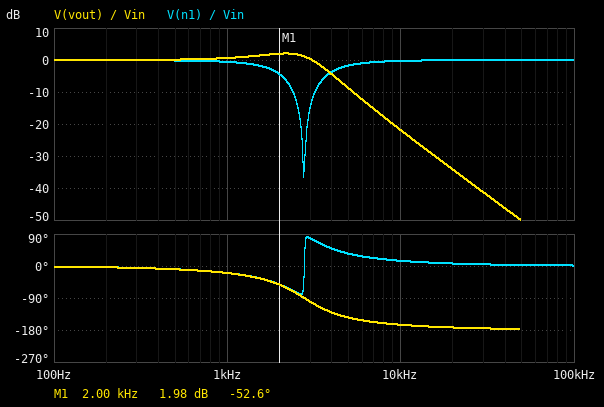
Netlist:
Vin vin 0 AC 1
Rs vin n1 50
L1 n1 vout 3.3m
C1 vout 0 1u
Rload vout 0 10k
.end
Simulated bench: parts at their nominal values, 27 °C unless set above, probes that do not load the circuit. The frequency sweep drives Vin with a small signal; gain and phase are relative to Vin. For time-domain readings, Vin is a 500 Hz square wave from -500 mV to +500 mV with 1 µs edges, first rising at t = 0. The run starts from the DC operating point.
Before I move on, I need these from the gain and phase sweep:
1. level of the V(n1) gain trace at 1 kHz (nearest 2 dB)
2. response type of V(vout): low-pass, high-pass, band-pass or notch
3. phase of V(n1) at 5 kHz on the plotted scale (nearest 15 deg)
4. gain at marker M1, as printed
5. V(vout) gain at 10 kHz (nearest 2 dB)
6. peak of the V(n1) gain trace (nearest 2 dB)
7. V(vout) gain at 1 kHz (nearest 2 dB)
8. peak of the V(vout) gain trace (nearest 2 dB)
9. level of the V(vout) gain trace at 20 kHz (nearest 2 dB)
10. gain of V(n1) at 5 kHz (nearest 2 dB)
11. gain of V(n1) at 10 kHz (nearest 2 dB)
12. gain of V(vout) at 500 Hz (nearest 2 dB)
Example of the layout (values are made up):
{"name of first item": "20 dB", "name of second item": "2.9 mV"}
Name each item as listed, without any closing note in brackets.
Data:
{"level of the V(n1) gain trace at 1 kHz": "0 dB", "response type of V(vout): low-pass, high-pass, band-pass or notch": "low-pass", "phase of V(n1) at 5 kHz on the plotted scale": "30 deg", "gain at marker M1, as printed": "1.98 dB", "V(vout) gain at 10 kHz": "-22 dB", "peak of the V(n1) gain trace": "0 dB", "V(vout) gain at 1 kHz": "0 dB", "peak of the V(vout) gain trace": "2 dB", "level of the V(vout) gain trace at 20 kHz": "-34 dB", "gain of V(n1) at 5 kHz": "-2 dB", "gain of V(n1) at 10 kHz": "0 dB", "gain of V(vout) at 500 Hz": "0 dB"}
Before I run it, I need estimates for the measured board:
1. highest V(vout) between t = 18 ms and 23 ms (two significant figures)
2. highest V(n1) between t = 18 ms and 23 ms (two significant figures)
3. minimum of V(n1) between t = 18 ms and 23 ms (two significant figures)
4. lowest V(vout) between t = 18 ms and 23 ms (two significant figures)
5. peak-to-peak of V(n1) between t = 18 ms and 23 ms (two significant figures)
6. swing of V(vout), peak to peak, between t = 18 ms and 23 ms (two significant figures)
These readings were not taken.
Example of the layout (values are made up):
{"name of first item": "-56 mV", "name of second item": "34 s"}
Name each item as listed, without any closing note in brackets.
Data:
{"highest V(vout) between t = 18 ms and 23 ms": "710 mV", "highest V(n1) between t = 18 ms and 23 ms": "610 mV", "minimum of V(n1) between t = 18 ms and 23 ms": "-610 mV", "lowest V(vout) between t = 18 ms and 23 ms": "-710 mV", "peak-to-peak of V(n1) between t = 18 ms and 23 ms": "1.2 V", "swing of V(vout), peak to peak, between t = 18 ms and 23 ms": "1.4 V"}
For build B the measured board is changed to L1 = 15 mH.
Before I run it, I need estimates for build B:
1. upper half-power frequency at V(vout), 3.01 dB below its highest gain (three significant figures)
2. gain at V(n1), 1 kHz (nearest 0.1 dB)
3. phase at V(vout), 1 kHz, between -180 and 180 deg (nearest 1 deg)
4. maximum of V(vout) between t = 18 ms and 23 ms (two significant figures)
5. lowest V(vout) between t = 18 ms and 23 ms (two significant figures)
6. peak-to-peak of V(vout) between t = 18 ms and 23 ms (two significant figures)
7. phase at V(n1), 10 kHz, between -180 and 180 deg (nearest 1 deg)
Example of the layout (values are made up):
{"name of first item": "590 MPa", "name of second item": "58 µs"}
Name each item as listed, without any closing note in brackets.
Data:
{"upper half-power frequency at V(vout), 3.01 dB below its highest gain": "1.50 kHz", "gain at V(n1), 1 kHz": "-2.2 dB", "phase at V(vout), 1 kHz, between -180 and 180 deg": "-38 deg", "maximum of V(vout) between t = 18 ms and 23 ms": "990 mV", "lowest V(vout) between t = 18 ms and 23 ms": "-990 mV", "peak-to-peak of V(vout) between t = 18 ms and 23 ms": "2.0 V", "phase at V(n1), 10 kHz, between -180 and 180 deg": "3 deg"}
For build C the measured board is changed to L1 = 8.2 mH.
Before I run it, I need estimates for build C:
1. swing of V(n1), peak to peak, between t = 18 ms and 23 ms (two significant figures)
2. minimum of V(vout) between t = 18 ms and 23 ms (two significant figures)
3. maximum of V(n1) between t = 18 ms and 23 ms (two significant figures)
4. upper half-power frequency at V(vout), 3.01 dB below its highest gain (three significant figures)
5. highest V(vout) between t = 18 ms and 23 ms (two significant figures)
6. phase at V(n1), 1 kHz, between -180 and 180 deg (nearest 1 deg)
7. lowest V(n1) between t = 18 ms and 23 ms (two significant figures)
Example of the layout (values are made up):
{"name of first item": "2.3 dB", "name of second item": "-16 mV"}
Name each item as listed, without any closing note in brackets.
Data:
{"swing of V(n1), peak to peak, between t = 18 ms and 23 ms": "1.3 V", "minimum of V(vout) between t = 18 ms and 23 ms": "-910 mV", "maximum of V(n1) between t = 18 ms and 23 ms": "650 mV", "upper half-power frequency at V(vout), 3.01 dB below its highest gain": "2.07 kHz", "highest V(vout) between t = 18 ms and 23 ms": "910 mV", "phase at V(n1), 1 kHz, between -180 and 180 deg": "-25 deg", "lowest V(n1) between t = 18 ms and 23 ms": "-650 mV"}
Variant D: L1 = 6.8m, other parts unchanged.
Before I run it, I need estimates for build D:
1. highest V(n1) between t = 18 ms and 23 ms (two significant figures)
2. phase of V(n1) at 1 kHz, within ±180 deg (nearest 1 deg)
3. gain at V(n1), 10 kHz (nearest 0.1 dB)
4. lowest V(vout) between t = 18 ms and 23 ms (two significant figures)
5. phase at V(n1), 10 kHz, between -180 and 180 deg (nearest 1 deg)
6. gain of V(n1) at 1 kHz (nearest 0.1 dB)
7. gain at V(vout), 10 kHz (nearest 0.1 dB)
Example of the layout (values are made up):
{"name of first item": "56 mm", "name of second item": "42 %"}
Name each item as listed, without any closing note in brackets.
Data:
{"highest V(n1) between t = 18 ms and 23 ms": "640 mV", "phase of V(n1) at 1 kHz, within ±180 deg": "-23 deg", "gain at V(n1), 10 kHz": "-0.1 dB", "lowest V(vout) between t = 18 ms and 23 ms": "-860 mV", "phase at V(n1), 10 kHz, between -180 and 180 deg": "7 deg", "gain of V(n1) at 1 kHz": "-0.8 dB", "gain at V(vout), 10 kHz": "-28.3 dB"}
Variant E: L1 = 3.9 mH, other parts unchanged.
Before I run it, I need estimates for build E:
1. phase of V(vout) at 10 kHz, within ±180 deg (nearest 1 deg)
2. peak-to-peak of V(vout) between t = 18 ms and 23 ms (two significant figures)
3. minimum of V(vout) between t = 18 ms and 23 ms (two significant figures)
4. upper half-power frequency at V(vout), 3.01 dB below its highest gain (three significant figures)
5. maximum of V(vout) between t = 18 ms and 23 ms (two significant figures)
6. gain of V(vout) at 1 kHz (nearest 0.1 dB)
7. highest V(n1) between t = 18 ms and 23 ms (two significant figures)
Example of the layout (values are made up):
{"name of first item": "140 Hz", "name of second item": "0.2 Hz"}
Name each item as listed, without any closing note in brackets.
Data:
{"phase of V(vout) at 10 kHz, within ±180 deg": "-168 deg", "peak-to-peak of V(vout) between t = 18 ms and 23 ms": "1.5 V", "minimum of V(vout) between t = 18 ms and 23 ms": "-750 mV", "upper half-power frequency at V(vout), 3.01 dB below its highest gain": "3.04 kHz", "maximum of V(vout) between t = 18 ms and 23 ms": "750 mV", "gain of V(vout) at 1 kHz": "0.8 dB", "highest V(n1) between t = 18 ms and 23 ms": "620 mV"}
